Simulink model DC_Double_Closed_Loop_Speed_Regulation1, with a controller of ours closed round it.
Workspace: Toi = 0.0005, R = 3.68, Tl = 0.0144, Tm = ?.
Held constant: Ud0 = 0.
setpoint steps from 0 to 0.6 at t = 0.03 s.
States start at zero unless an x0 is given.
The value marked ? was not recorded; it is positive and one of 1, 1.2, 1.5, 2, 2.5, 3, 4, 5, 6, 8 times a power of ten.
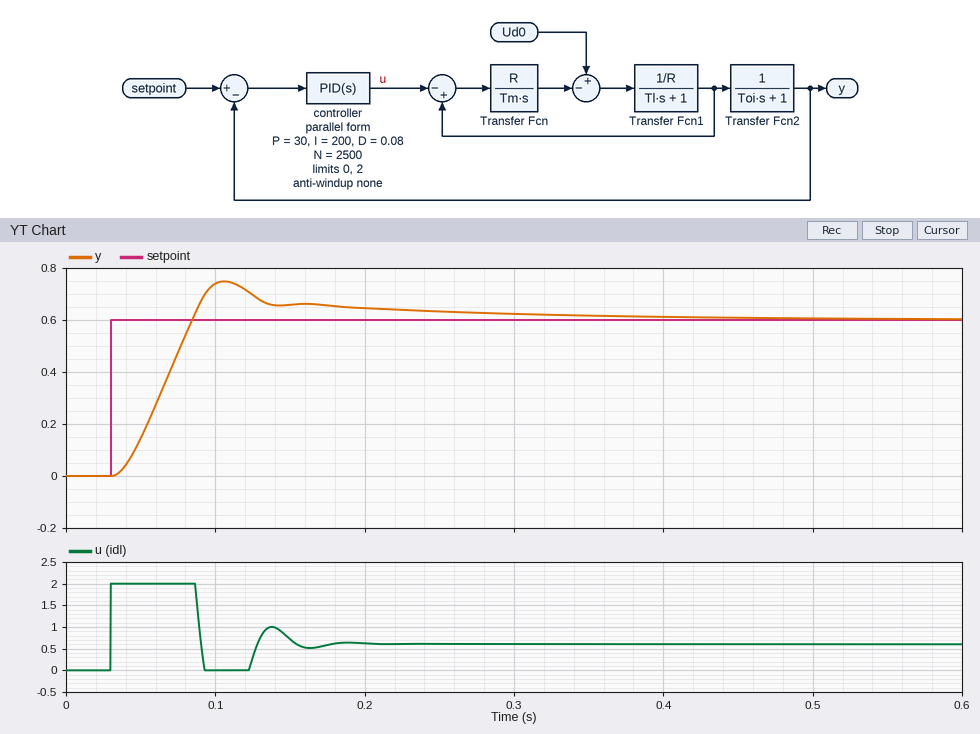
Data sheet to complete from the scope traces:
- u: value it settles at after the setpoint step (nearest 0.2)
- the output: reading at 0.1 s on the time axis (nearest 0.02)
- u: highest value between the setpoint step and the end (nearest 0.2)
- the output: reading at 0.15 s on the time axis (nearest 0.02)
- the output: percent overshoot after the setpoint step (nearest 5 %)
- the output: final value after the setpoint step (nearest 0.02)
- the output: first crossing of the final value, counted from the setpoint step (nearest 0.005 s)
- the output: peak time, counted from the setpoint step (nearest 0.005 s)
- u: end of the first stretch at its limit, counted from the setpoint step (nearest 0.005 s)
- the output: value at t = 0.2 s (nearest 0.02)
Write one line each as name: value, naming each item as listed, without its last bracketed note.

u: value it settles at after the setpoint step: 0.6
the output: reading at 0.1 s on the time axis: 0.74
u: highest value between the setpoint step and the end: 2.0
the output: reading at 0.15 s on the time axis: 0.66
the output: percent overshoot after the setpoint step: 25 %
the output: final value after the setpoint step: 0.60
the output: first crossing of the final value, counted from the setpoint step: 0.055 s
the output: peak time, counted from the setpoint step: 0.075 s
u: end of the first stretch at its limit, counted from the setpoint step: 0.055 s
the output: value at t = 0.2 s: 0.64
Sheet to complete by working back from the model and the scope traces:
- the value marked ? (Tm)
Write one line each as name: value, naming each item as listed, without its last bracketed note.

the value marked ?: 0.12
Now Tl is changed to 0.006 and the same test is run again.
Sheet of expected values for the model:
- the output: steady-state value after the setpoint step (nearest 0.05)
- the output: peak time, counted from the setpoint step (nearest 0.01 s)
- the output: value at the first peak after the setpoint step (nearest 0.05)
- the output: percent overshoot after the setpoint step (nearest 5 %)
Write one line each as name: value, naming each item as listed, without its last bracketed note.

the output: steady-state value after the setpoint step: 0.60
the output: peak time, counted from the setpoint step: 0.06 s
the output: value at the first peak after the setpoint step: 0.70
the output: percent overshoot after the setpoint step: 15 %
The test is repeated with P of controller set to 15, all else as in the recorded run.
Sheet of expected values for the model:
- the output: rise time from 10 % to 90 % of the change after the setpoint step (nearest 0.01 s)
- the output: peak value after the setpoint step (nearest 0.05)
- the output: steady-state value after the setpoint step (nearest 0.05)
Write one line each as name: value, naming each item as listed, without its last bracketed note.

the output: rise time from 10 % to 90 % of the change after the setpoint step: 0.04 s
the output: peak value after the setpoint step: 0.80
the output: steady-state value after the setpoint step: 0.60
